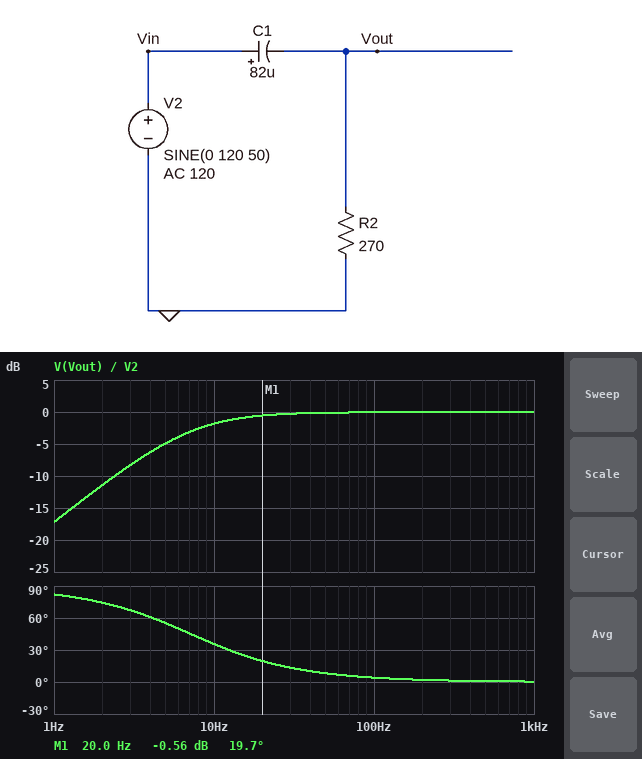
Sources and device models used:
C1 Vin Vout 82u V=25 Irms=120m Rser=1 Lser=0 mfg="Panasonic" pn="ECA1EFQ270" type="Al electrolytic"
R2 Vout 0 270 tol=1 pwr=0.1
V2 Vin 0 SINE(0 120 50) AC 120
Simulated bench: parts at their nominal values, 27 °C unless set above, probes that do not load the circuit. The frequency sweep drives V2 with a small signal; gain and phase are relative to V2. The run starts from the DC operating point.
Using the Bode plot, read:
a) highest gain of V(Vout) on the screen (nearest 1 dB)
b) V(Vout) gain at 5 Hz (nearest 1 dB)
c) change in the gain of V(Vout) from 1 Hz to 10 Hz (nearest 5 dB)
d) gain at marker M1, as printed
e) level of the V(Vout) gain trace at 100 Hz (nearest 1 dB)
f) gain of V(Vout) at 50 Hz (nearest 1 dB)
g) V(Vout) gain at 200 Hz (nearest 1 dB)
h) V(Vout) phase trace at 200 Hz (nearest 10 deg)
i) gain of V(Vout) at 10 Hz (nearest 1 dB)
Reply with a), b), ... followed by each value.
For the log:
a) 0 dB
b) -5 dB
c) 15 dB
d) -0.56 dB
e) 0 dB
f) 0 dB
g) 0 dB
h) 0 deg
i) -2 dB
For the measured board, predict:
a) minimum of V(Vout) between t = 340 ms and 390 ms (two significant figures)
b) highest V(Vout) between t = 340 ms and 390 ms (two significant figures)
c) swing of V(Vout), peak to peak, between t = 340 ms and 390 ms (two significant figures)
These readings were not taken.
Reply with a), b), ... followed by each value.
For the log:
a) -120 V
b) 120 V
c) 240 V
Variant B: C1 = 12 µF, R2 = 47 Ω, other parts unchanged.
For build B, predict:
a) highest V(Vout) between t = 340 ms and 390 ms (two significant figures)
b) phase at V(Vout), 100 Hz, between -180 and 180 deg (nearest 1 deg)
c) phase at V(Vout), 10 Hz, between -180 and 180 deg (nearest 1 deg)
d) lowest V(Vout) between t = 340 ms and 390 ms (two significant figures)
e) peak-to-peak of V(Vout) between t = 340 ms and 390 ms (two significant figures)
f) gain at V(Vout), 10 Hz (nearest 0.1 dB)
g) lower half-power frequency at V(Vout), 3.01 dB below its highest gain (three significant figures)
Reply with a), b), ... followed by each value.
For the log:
a) 21 V
b) 70 deg
c) 88 deg
d) -21 V
e) 42 V
f) -29.0 dB
g) 276 Hz
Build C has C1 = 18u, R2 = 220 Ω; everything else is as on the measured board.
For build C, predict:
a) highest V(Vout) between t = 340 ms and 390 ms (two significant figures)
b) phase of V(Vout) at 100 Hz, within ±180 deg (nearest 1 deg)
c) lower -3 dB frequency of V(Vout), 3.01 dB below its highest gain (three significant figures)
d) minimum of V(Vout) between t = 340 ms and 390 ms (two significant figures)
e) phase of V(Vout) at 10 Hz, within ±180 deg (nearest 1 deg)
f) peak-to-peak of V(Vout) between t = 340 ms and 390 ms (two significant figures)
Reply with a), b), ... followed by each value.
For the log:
a) 93 V
b) 22 deg
c) 40.0 Hz
d) -93 V
e) 76 deg
f) 190 V
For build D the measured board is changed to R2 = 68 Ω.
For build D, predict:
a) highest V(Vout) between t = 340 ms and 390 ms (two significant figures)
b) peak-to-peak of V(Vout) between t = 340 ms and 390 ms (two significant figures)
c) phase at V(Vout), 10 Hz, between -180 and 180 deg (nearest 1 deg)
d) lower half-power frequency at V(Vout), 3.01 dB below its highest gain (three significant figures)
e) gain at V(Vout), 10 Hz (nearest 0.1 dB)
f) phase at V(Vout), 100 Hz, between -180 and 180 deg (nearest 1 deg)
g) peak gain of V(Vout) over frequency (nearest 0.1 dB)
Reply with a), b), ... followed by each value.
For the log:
a) 100 V
b) 210 V
c) 70 deg
d) 28.1 Hz
e) -9.6 dB
f) 16 deg
g) -0.1 dB
